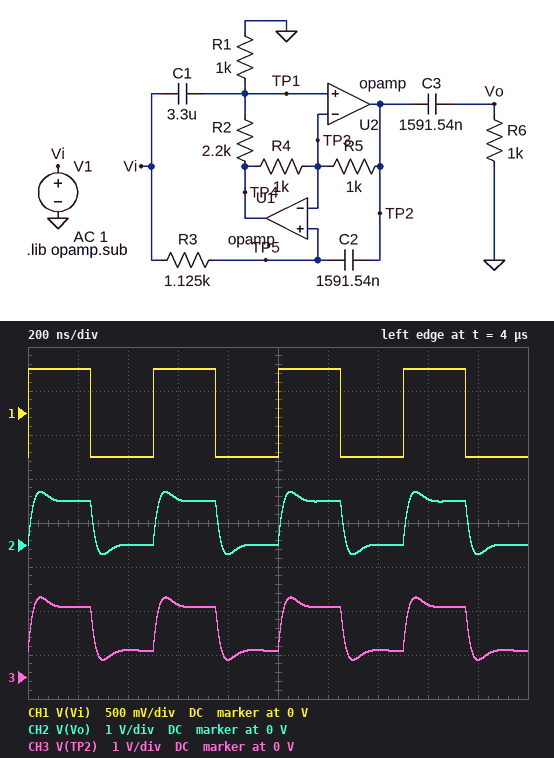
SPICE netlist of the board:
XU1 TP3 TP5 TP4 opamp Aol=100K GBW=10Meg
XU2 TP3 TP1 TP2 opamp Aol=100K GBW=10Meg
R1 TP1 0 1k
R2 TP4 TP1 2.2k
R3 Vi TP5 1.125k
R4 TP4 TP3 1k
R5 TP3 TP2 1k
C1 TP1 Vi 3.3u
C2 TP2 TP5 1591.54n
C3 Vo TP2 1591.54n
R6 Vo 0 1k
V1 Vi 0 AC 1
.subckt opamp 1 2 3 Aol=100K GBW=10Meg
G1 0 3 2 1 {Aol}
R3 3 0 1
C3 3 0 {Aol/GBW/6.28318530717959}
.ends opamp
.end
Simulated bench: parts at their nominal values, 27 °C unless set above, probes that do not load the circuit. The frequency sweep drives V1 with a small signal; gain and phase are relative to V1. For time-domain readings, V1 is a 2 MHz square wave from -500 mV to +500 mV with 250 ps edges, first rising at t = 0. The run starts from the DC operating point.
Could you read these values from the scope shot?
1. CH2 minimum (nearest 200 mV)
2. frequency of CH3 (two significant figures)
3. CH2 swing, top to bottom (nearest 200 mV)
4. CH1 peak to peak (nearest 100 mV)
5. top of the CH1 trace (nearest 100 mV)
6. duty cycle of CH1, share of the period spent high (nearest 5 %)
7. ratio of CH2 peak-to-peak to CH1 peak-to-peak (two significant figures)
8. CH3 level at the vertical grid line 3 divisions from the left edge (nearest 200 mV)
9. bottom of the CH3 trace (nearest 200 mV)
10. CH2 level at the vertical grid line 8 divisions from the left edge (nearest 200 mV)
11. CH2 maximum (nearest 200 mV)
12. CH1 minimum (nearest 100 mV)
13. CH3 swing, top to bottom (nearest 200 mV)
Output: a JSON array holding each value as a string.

["-200 mV", "2.0 MHz", "1.4 V", "1.0 V", "500 mV", "50 %", "1.4", "1.6 V", "400 mV", "1.0 V", "1.2 V", "-500 mV", "1.4 V"]
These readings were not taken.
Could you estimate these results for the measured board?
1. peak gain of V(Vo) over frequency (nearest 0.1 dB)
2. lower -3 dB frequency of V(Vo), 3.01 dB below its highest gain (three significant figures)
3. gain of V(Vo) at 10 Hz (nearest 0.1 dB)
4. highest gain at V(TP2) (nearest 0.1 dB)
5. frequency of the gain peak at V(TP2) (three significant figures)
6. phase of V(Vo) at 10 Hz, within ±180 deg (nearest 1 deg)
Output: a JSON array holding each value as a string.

["0 dB", "38.0 Hz", "-17.9 dB", "6.1 dB", "42.5 Hz", "-110 deg"]
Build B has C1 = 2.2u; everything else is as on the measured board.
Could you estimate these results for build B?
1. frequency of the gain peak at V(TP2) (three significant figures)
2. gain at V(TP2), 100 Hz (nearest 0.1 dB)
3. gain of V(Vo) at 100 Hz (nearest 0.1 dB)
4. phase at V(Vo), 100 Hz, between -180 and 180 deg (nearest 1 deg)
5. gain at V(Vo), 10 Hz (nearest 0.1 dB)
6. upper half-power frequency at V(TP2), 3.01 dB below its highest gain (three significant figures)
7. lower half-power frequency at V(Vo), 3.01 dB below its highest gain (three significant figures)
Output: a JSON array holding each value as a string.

["50.2 Hz", "2.5 dB", "-0.5 dB", "91 deg", "-18.2 dB", "148 Hz", "47.6 Hz"]
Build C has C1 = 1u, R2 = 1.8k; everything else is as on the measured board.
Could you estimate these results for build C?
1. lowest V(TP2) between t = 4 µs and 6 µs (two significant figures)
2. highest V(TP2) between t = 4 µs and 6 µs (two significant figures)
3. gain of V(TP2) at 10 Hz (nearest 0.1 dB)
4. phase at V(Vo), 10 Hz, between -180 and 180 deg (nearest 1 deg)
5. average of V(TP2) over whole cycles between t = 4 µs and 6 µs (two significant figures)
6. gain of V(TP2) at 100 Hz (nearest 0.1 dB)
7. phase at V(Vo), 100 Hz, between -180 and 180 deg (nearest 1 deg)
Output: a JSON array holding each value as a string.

["190 mV", "1.6 V", "-1.9 dB", "-107 deg", "900 mV", "0.1 dB", "127 deg"]
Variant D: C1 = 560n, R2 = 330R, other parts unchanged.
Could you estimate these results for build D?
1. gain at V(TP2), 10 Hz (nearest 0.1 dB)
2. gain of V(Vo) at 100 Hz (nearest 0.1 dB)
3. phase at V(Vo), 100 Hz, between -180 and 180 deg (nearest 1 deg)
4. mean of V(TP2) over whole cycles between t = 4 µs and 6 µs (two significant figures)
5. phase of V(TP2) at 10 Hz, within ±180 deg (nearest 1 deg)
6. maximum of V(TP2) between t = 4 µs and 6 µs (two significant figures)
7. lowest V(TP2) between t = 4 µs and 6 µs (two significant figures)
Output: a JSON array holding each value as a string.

["-3.5 dB", "-7.9 dB", "22 deg", "160 mV", "-2 deg", "870 mV", "-550 mV"]
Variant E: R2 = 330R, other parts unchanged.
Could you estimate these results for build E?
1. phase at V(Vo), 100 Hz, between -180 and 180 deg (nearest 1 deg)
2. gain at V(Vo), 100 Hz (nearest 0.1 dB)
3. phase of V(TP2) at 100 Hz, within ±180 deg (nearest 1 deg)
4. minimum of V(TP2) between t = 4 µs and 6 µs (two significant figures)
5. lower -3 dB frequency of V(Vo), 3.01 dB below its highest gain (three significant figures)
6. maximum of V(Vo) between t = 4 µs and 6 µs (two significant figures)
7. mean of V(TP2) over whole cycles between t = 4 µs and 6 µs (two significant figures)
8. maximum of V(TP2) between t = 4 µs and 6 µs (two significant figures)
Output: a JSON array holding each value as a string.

["167 deg", "-15.8 dB", "122 deg", "-540 mV", "119 Hz", "1.2 V", "160 mV", "870 mV"]
